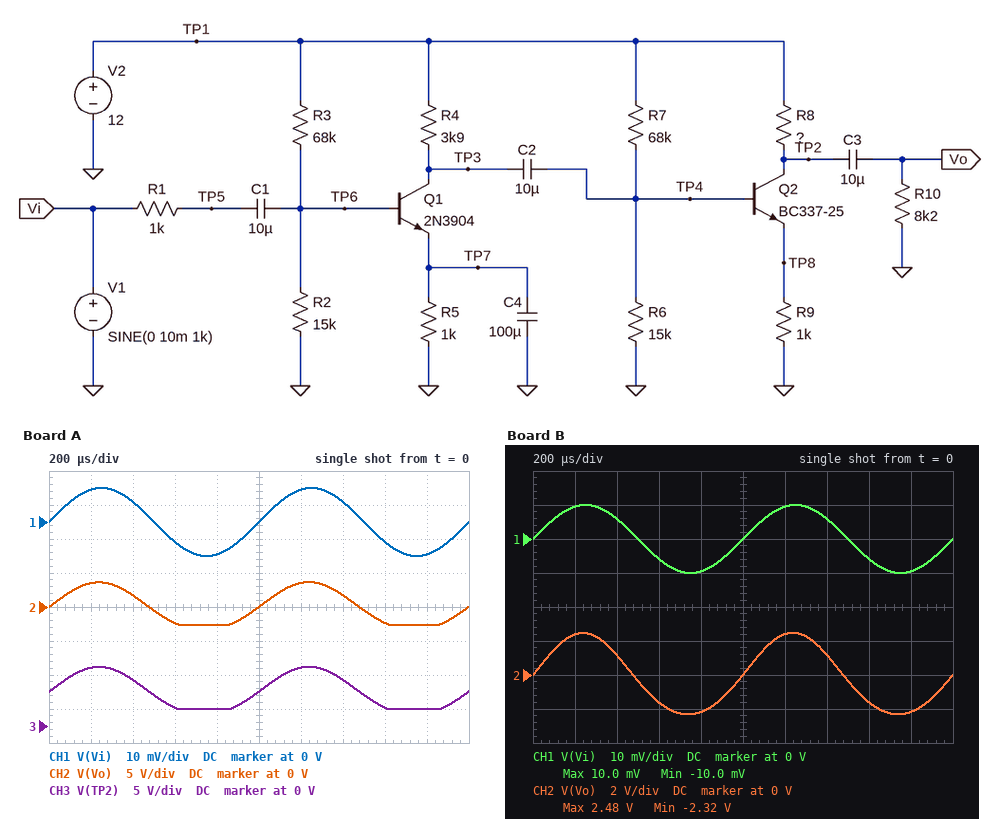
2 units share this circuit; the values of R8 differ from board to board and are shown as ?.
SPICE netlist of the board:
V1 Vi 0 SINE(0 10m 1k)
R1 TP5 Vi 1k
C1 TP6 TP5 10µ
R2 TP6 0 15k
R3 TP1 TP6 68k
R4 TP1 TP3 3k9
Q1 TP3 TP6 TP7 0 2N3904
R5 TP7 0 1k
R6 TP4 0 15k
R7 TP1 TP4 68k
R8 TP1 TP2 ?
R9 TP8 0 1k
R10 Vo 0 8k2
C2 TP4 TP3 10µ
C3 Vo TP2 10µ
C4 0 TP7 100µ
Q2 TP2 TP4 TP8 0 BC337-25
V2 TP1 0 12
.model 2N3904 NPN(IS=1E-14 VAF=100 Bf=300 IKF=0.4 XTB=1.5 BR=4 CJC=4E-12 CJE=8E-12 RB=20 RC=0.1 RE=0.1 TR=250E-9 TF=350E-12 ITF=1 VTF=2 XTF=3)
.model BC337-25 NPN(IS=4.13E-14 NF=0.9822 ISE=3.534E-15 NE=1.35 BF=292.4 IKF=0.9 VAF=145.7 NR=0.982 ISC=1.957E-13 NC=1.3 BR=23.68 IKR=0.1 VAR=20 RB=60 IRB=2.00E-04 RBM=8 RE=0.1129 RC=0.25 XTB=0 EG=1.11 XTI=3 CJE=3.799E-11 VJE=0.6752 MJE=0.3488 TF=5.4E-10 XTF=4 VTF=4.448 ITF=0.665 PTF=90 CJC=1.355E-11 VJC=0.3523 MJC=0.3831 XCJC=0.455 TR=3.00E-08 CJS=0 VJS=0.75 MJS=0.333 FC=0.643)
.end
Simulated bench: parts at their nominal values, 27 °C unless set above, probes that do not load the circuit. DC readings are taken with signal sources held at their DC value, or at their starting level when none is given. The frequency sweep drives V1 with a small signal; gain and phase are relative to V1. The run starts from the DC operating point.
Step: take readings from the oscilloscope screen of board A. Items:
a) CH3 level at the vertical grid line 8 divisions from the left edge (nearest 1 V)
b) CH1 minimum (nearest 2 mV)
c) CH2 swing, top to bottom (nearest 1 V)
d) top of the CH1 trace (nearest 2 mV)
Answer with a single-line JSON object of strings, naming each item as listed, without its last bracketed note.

{"CH3 level at the vertical grid line 8 divisions from the left edge": "3 V", "CH1 minimum": "-10 mV", "CH2 swing, top to bottom": "6 V", "top of the CH1 trace": "10 mV"}
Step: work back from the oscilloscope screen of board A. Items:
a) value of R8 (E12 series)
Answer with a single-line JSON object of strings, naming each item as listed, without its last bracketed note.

{"value of R8": "4.7 kΩ"}
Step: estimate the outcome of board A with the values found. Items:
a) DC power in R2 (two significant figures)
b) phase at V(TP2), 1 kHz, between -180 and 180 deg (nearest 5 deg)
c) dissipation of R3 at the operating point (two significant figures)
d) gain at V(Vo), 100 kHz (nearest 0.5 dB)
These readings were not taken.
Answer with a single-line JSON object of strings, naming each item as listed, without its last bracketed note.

{"DC power in R2": "300 µW", "phase at V(TP2), 1 kHz, between -180 and 180 deg": "5 deg", "dissipation of R3 at the operating point": "1.4 mW", "gain at V(Vo), 100 kHz": "51.0 dB"}
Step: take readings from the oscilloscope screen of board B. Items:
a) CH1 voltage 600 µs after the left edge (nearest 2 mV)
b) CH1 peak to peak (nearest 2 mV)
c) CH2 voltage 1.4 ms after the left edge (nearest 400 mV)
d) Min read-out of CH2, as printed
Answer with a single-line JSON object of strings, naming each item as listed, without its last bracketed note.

{"CH1 voltage 600 µs after the left edge": "-6 mV", "CH1 peak to peak": "20 mV", "CH2 voltage 1.4 ms after the left edge": "1.2 V", "Min read-out of CH2, as printed": "-2.32 V"}
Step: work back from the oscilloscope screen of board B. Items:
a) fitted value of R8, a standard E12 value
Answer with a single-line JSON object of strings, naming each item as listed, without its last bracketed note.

{"fitted value of R8, a standard E12 value": "2.7 kΩ"}
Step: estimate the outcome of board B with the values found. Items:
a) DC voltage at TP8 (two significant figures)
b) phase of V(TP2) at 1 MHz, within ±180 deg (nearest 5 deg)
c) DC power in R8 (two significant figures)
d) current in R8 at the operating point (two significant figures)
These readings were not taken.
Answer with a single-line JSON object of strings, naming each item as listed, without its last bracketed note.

{"DC voltage at TP8": "1.5 V", "phase of V(TP2) at 1 MHz, within ±180 deg": "-70 deg", "DC power in R8": "5.9 mW", "current in R8 at the operating point": "1.5 mA"}
